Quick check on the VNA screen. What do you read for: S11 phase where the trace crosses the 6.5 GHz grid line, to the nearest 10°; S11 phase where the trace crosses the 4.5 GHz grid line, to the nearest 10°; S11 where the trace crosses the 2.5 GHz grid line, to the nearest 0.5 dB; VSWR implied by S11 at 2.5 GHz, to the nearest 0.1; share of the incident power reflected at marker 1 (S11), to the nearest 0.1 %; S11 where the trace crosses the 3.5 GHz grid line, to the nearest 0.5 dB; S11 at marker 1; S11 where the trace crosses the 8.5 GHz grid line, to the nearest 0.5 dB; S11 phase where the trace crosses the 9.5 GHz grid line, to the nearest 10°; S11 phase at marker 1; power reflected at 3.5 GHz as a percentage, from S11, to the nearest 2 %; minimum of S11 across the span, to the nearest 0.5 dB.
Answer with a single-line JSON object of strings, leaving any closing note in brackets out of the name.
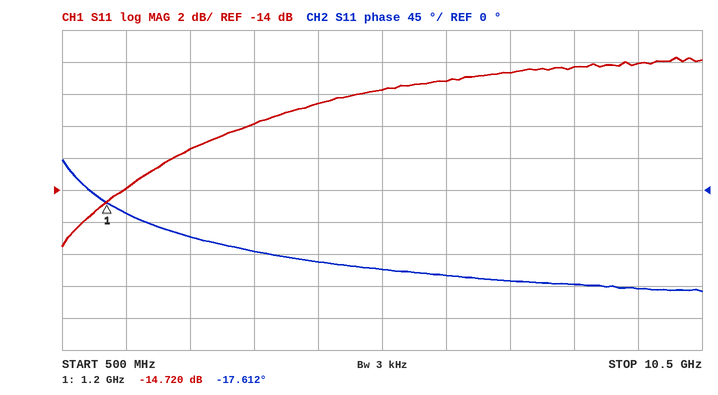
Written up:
{"S11 phase where the trace crosses the 6.5 GHz grid line, to the nearest 10°": "-120°", "S11 phase where the trace crosses the 4.5 GHz grid line, to the nearest 10°": "-100°", "S11 where the trace crosses the 2.5 GHz grid line, to the nearest 0.5 dB": "-11.5 dB", "VSWR implied by S11 at 2.5 GHz, to the nearest 0.1": "1.7", "share of the incident power reflected at marker 1 (S11), to the nearest 0.1 %": "3.4 %", "S11 where the trace crosses the 3.5 GHz grid line, to the nearest 0.5 dB": "-10.0 dB", "S11 at marker 1": "-14.720 dB", "S11 where the trace crosses the 8.5 GHz grid line, to the nearest 0.5 dB": "-6.5 dB", "S11 phase where the trace crosses the 9.5 GHz grid line, to the nearest 10°": "-140°", "S11 phase at marker 1": "-17.612°", "power reflected at 3.5 GHz as a percentage, from S11, to the nearest 2 %": "10 %", "minimum of S11 across the span, to the nearest 0.5 dB": "-17.5 dB"}
